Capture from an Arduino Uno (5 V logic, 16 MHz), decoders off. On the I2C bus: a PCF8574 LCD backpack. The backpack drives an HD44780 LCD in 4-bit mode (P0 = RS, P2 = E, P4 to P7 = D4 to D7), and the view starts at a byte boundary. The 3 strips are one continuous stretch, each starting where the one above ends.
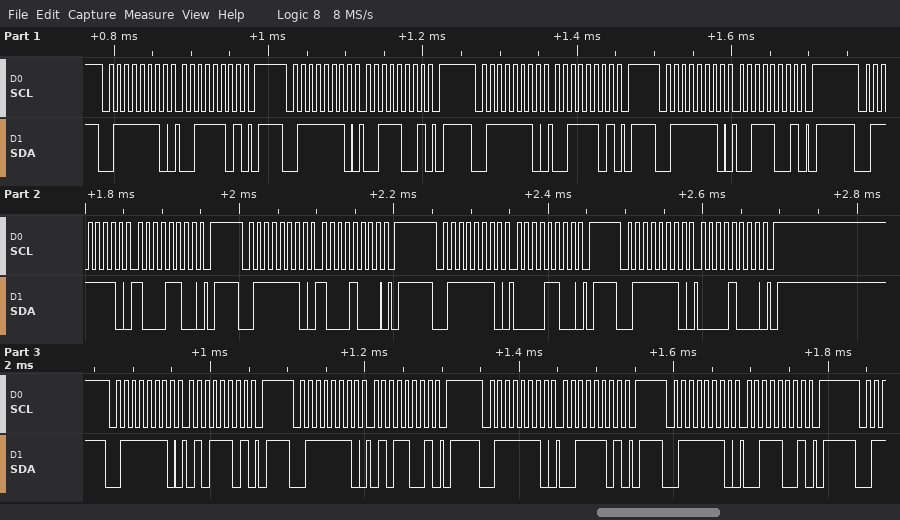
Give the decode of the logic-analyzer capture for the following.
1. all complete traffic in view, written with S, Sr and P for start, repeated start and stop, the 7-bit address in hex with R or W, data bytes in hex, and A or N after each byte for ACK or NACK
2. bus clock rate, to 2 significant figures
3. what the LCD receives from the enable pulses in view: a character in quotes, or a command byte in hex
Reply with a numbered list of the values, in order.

1. S 3FW A 3D A P S 3FW A 39 A P S 3FW A 3D A P S 3FW A 39 A P S 3FW A 8C A P S 3FW A 88 A P S 3FW A 0C A P S 3FW A 08 A P S 3FW A 5D A P S 3FW A 59 A P S 3FW A 3D A P S 3FW A 39 A P
2. 100 kHz
3. '3' 0x80 'S'
